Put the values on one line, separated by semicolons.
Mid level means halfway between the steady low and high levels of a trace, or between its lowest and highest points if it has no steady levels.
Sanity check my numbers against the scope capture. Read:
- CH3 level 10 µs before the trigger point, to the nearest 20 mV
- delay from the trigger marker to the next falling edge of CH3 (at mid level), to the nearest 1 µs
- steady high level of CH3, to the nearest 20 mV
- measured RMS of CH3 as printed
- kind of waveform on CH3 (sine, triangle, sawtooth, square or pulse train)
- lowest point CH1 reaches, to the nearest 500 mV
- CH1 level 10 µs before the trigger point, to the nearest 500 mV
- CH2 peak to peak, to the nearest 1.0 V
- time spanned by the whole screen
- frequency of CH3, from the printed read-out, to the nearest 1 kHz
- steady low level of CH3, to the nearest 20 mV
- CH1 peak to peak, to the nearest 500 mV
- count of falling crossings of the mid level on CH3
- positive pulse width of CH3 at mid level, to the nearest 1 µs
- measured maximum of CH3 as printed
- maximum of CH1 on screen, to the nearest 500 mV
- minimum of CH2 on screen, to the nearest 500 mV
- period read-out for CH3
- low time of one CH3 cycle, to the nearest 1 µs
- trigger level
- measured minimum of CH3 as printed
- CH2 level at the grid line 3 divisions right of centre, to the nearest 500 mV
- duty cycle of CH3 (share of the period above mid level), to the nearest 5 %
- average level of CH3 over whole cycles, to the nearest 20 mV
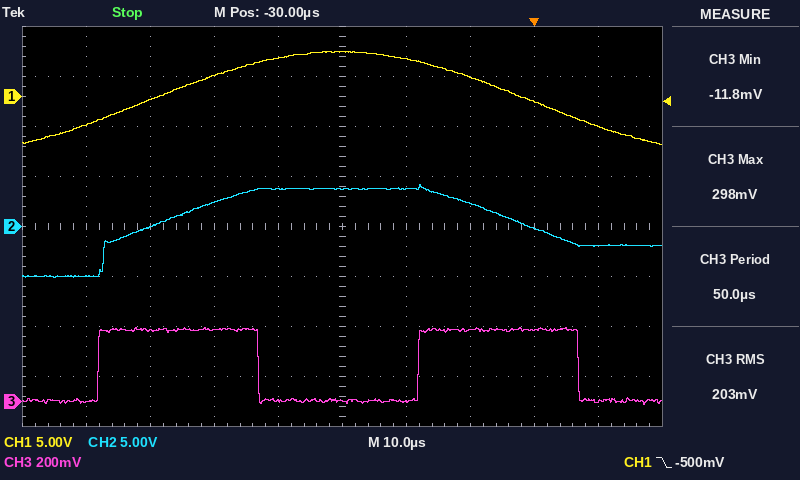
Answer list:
280 mV; 7 µs; 280 mV; 203 mV; square; -5.0 V; 2.0 V; 9.0 V; 100 µs; 20 kHz; 0 mV; 9.5 V; 2; 25 µs; 298 mV; 4.5 V; -5.0 V; 50.0 µs; 25 µs; -500 mV; -11.8 mV; 0.0 V; 50 %; 140 mV
